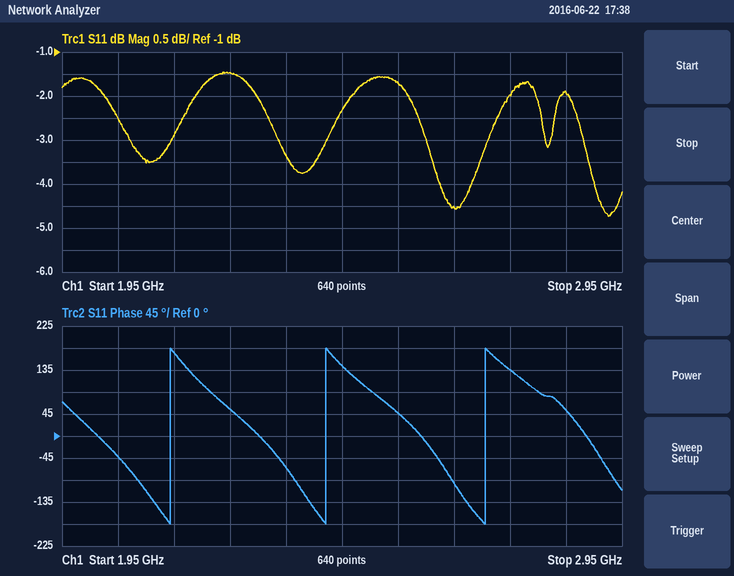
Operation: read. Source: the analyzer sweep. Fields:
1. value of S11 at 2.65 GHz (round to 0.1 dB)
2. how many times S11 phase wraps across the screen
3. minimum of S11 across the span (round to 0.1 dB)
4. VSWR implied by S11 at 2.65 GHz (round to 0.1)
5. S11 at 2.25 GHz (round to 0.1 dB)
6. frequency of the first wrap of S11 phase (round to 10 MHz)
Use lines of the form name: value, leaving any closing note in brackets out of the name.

value of S11 at 2.65 GHz: -4.5 dB
how many times S11 phase wraps across the screen: 3
minimum of S11 across the span: -4.7 dB
VSWR implied by S11 at 2.65 GHz: 3.9
S11 at 2.25 GHz: -1.5 dB
frequency of the first wrap of S11 phase: 2.14 GHz
